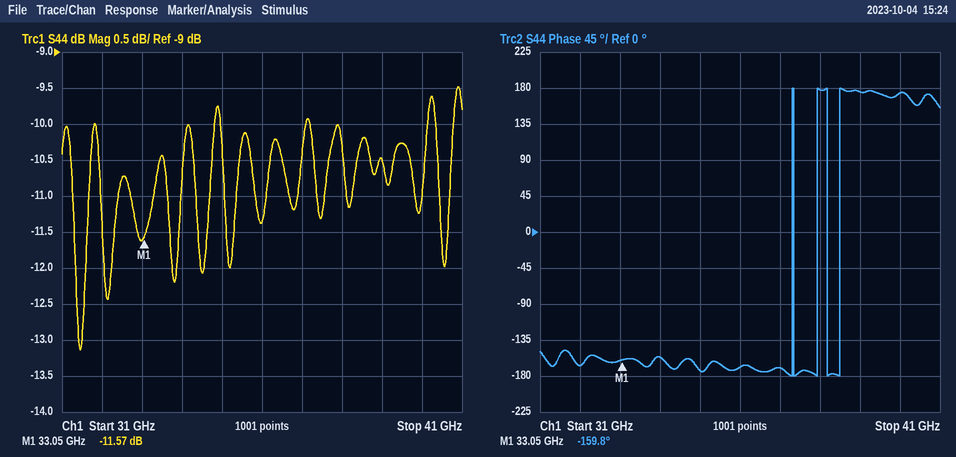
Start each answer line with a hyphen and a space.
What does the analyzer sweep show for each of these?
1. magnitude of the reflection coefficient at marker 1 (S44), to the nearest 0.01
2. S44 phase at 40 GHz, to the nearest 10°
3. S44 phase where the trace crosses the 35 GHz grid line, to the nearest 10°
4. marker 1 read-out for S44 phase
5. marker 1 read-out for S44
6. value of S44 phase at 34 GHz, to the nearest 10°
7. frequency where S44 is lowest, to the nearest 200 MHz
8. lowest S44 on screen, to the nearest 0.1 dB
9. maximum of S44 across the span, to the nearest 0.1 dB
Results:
- 0.26
- 170°
- -170°
- -159.8°
- -11.57 dB
- -160°
- 31.4 GHz
- -13.1 dB
- -9.5 dB
